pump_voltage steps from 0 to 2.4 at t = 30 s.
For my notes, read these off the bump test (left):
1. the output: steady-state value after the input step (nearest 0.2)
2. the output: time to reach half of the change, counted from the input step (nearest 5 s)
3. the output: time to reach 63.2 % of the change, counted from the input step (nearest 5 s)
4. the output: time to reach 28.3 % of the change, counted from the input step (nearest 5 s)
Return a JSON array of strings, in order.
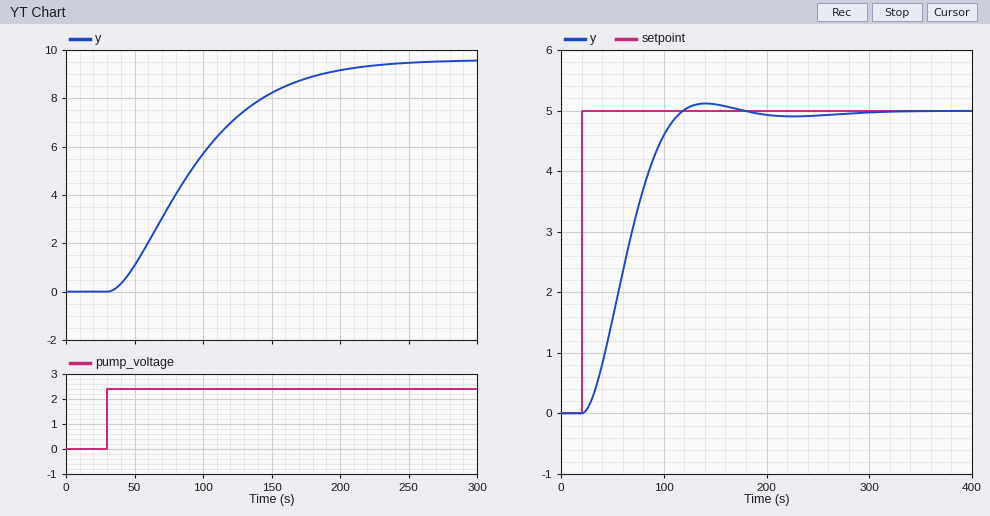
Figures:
["9.6", "60 s", "75 s", "35 s"]
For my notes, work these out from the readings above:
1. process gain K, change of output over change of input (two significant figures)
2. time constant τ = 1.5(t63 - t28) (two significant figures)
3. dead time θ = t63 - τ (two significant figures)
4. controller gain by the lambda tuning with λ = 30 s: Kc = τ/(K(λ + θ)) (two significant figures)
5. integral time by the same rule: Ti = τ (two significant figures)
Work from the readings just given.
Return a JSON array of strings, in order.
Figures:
["4.0", "60 s", "15 s", "0.33", "60 s"]
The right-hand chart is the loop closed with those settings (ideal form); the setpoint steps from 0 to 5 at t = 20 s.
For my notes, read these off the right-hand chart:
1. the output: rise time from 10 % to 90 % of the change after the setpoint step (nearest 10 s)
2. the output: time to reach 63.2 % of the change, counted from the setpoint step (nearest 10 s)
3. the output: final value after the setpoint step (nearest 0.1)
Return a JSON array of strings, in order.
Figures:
["60 s", "50 s", "5.0"]
